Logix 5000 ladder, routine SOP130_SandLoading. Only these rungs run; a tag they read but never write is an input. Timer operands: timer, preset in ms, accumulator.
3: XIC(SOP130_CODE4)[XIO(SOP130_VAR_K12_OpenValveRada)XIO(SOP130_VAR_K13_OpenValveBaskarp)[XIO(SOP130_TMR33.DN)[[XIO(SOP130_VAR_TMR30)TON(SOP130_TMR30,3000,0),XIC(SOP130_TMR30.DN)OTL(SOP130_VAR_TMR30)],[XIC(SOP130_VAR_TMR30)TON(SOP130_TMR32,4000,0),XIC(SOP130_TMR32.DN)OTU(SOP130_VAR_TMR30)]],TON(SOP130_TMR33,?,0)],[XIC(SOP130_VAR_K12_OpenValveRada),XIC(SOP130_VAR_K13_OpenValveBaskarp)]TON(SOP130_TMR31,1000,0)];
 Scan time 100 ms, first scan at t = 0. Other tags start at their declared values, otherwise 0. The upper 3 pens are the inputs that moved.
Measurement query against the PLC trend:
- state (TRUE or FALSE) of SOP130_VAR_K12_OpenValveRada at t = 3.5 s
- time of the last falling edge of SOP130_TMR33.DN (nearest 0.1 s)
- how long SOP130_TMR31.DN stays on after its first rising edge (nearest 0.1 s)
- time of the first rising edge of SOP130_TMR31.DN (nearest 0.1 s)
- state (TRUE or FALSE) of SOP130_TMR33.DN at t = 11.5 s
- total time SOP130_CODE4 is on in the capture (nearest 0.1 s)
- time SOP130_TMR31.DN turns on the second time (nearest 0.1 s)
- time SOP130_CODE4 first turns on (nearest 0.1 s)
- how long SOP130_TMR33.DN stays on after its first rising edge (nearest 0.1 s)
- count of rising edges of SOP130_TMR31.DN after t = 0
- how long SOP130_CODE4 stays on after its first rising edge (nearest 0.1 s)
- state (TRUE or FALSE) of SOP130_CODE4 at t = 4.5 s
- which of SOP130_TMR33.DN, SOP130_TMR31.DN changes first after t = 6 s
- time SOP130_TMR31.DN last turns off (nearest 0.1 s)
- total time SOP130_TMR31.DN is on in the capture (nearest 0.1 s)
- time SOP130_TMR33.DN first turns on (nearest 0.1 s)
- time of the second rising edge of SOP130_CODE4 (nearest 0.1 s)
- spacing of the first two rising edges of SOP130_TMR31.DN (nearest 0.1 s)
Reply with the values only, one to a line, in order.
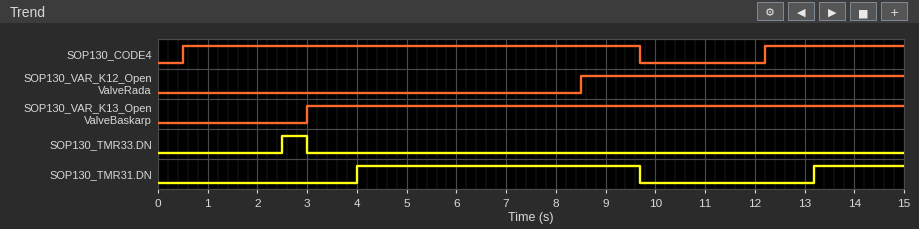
FALSE
3.0 s
5.7 s
4.0 s
FALSE
12.0 s
13.2 s
0.5 s
0.5 s
2
9.2 s
TRUE
SOP130_TMR31.DN
9.7 s
7.5 s
2.5 s
12.2 s
9.2 s
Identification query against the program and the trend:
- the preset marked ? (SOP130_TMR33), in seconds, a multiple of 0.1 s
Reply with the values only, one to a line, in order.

2.0 s
